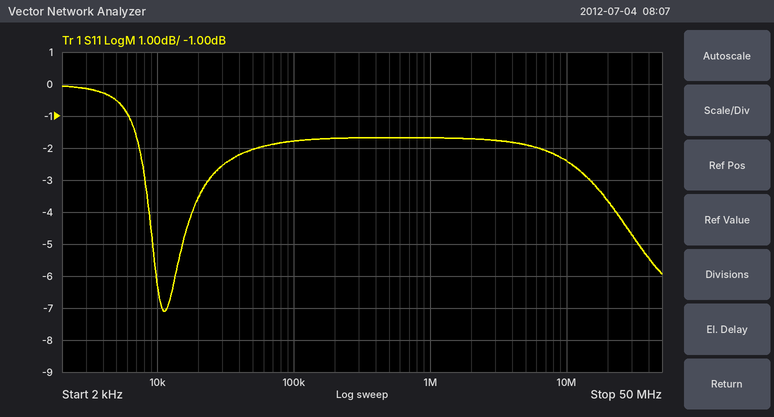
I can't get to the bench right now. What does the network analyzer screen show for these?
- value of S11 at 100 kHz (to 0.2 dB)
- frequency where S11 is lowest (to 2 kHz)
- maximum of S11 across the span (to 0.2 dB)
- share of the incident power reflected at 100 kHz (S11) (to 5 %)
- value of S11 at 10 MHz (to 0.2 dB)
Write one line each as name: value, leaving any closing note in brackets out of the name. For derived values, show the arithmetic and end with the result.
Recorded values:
value of S11 at 100 kHz: -1.8 dB
frequency where S11 is lowest: 12 kHz
maximum of S11 across the span: 0.0 dB
share of the incident power reflected at 100 kHz (S11): 10^(-1.8/10) ≈ 66.1 %, so 65 % to the nearest 5 %
value of S11 at 10 MHz: -2.4 dB
